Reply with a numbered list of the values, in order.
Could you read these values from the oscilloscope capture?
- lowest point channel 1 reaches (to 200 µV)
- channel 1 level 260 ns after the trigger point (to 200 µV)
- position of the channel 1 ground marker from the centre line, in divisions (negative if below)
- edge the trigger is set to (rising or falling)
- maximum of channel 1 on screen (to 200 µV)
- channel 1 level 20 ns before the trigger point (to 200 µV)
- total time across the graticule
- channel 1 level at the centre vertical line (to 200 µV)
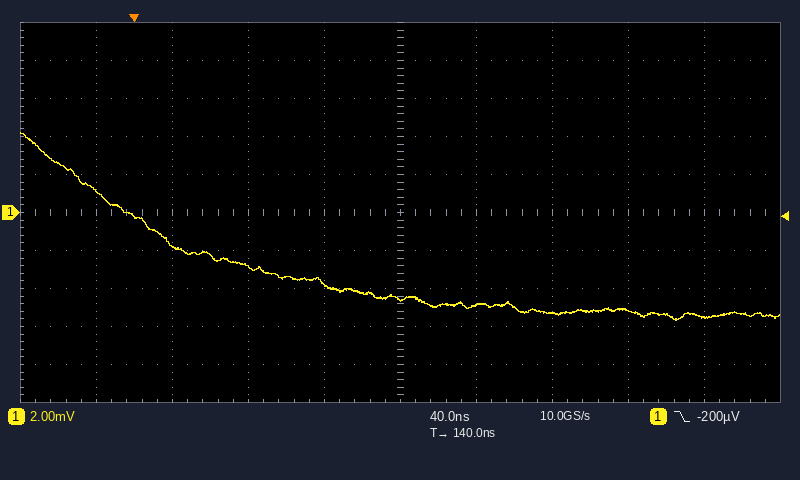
1. -5.6 mV
2. -5.2 mV
3. 0.0 div
4. falling
5. 4.2 mV
6. 1.2 mV
7. 400 ns
8. -4.6 mV
